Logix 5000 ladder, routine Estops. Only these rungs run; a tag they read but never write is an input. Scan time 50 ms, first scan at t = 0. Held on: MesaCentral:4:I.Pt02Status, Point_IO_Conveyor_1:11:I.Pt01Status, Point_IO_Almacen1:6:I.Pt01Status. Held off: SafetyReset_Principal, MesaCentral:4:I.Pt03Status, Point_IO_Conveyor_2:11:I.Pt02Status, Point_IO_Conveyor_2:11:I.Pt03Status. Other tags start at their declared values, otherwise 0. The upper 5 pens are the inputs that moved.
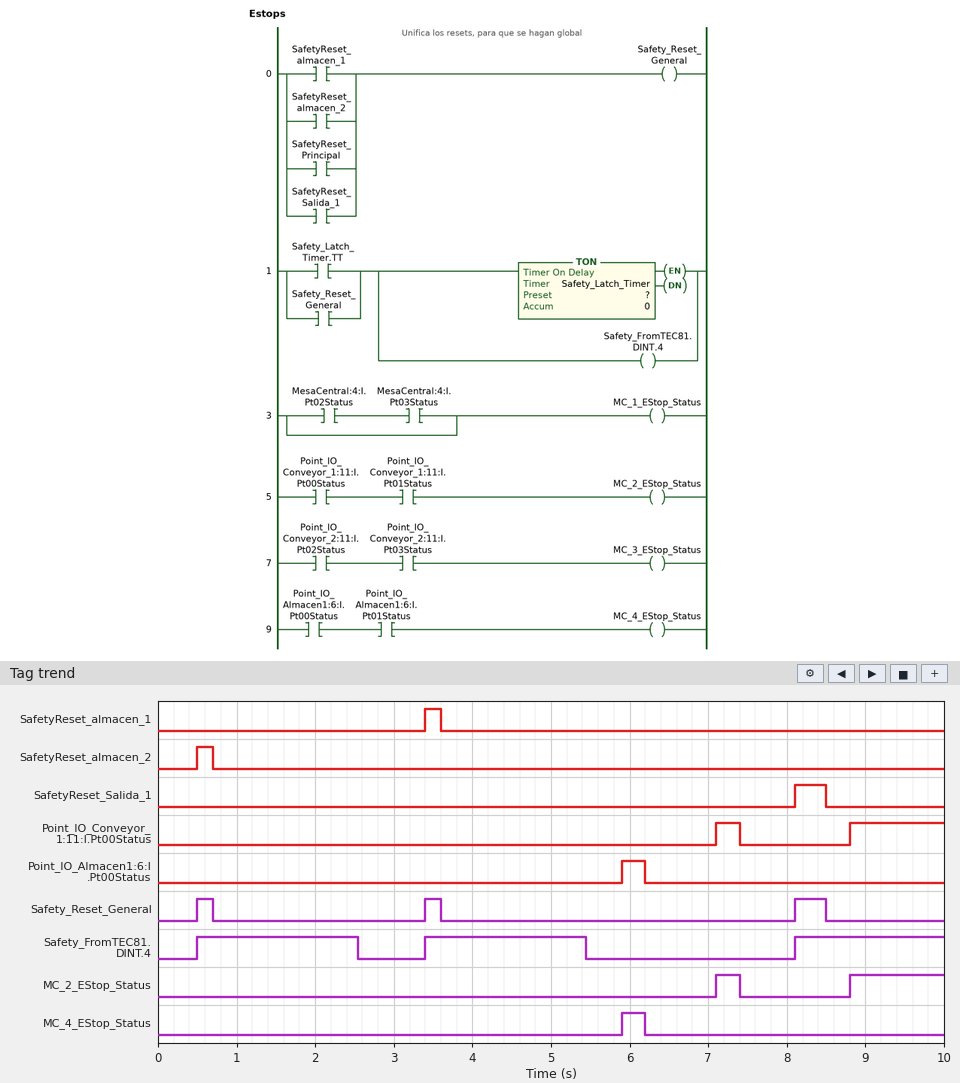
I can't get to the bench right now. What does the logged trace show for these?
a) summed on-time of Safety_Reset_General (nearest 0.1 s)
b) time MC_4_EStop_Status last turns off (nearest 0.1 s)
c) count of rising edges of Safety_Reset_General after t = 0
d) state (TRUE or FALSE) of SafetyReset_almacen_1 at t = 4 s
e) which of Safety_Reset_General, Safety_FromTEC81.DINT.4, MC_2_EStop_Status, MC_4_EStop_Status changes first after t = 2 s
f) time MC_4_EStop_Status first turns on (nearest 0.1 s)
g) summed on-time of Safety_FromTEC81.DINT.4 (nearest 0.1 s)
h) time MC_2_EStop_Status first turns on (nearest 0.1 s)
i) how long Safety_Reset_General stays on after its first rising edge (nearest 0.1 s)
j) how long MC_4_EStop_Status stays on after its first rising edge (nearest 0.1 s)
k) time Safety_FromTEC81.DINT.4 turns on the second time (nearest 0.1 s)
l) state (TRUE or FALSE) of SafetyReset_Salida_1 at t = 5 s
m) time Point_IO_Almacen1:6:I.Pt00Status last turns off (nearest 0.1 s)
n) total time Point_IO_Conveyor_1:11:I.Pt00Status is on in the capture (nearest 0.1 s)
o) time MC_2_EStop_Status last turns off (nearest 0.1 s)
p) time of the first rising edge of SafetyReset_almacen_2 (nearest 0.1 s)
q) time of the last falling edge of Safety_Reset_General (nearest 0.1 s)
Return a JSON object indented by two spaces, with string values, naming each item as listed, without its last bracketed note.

{
  "summed on-time of Safety_Reset_General": "0.8 s",
  "time MC_4_EStop_Status last turns off": "6.2 s",
  "count of rising edges of Safety_Reset_General after t = 0": "3",
  "state (TRUE or FALSE) of SafetyReset_almacen_1 at t = 4 s": "FALSE",
  "which of Safety_Reset_General, Safety_FromTEC81.DINT.4, MC_2_EStop_Status, MC_4_EStop_Status changes first after t = 2 s": "Safety_FromTEC81.DINT.4",
  "time MC_4_EStop_Status first turns on": "5.9 s",
  "summed on-time of Safety_FromTEC81.DINT.4": "6.0 s",
  "time MC_2_EStop_Status first turns on": "7.1 s",
  "how long Safety_Reset_General stays on after its first rising edge": "0.2 s",
  "how long MC_4_EStop_Status stays on after its first rising edge": "0.3 s",
  "time Safety_FromTEC81.DINT.4 turns on the second time": "3.4 s",
  "state (TRUE or FALSE) of SafetyReset_Salida_1 at t = 5 s": "FALSE",
  "time Point_IO_Almacen1:6:I.Pt00Status last turns off": "6.2 s",
  "total time Point_IO_Conveyor_1:11:I.Pt00Status is on in the capture": "1.5 s",
  "time MC_2_EStop_Status last turns off": "7.4 s",
  "time of the first rising edge of SafetyReset_almacen_2": "0.5 s",
  "time of the last falling edge of Safety_Reset_General": "8.5 s"
}
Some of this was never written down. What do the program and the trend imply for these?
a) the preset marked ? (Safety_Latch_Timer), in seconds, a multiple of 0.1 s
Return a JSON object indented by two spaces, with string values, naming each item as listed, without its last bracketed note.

{
  "the preset marked ? (Safety_Latch_Timer), in seconds, a multiple of 0.1 s": "2.0 s"
}
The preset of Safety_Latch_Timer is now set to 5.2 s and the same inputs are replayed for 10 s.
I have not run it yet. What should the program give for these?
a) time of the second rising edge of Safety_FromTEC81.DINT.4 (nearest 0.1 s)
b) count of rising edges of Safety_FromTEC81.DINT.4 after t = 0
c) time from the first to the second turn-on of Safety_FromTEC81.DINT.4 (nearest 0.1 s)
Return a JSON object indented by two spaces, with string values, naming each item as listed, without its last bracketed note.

{
  "time of the second rising edge of Safety_FromTEC81.DINT.4": "8.1 s",
  "count of rising edges of Safety_FromTEC81.DINT.4 after t = 0": "2",
  "time from the first to the second turn-on of Safety_FromTEC81.DINT.4": "7.6 s"
}
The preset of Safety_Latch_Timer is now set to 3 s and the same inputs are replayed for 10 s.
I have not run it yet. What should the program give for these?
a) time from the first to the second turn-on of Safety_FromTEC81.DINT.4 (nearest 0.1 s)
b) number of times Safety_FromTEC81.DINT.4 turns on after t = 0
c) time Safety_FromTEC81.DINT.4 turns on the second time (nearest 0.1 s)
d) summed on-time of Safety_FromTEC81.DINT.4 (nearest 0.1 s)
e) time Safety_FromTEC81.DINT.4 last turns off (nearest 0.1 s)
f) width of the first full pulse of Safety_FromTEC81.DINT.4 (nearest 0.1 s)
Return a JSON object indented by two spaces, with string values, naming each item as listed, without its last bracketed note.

{
  "time from the first to the second turn-on of Safety_FromTEC81.DINT.4": "7.6 s",
  "number of times Safety_FromTEC81.DINT.4 turns on after t = 0": "2",
  "time Safety_FromTEC81.DINT.4 turns on the second time": "8.1 s",
  "summed on-time of Safety_FromTEC81.DINT.4": "5.0 s",
  "time Safety_FromTEC81.DINT.4 last turns off": "3.6 s",
  "width of the first full pulse of Safety_FromTEC81.DINT.4": "3.1 s"
}
